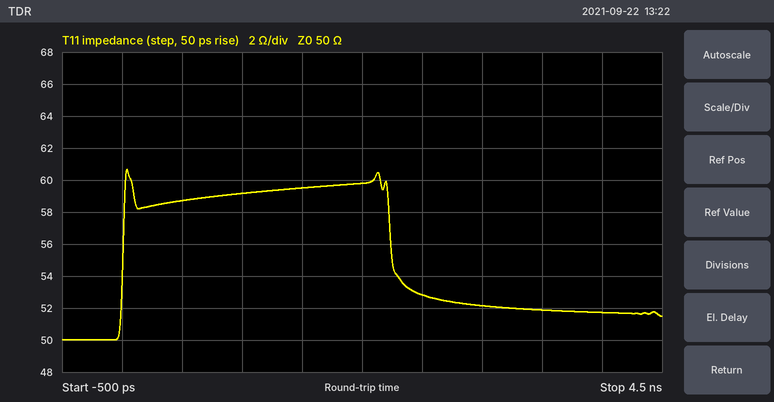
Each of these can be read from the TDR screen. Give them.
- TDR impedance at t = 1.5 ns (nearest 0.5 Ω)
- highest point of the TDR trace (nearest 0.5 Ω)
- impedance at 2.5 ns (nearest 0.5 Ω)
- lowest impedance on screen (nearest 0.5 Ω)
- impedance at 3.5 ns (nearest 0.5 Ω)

59.5 Ω
60.5 Ω
53.0 Ω
50.0 Ω
52.0 Ω
